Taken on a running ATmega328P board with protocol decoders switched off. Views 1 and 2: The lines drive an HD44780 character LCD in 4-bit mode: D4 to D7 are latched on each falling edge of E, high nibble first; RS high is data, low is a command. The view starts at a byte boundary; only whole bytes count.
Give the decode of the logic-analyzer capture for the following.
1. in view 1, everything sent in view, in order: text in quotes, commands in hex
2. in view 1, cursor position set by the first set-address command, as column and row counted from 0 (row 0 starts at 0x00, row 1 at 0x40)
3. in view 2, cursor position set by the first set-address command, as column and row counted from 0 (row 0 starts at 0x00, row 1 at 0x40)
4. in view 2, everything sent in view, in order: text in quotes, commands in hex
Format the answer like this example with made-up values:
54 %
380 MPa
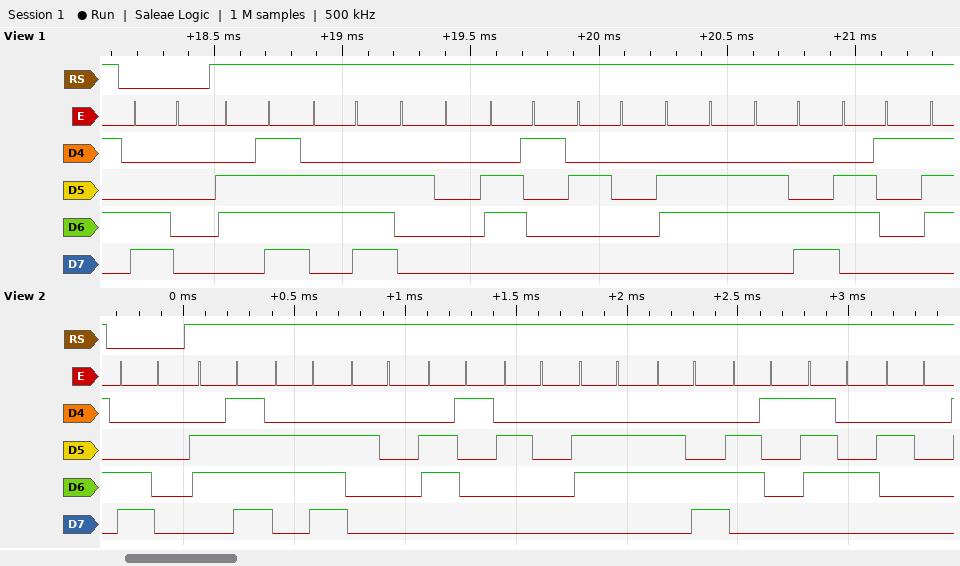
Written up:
0xC0 "on a fla"
column 0, row 1
column 0, row 1
0xC0 "on a flat "
